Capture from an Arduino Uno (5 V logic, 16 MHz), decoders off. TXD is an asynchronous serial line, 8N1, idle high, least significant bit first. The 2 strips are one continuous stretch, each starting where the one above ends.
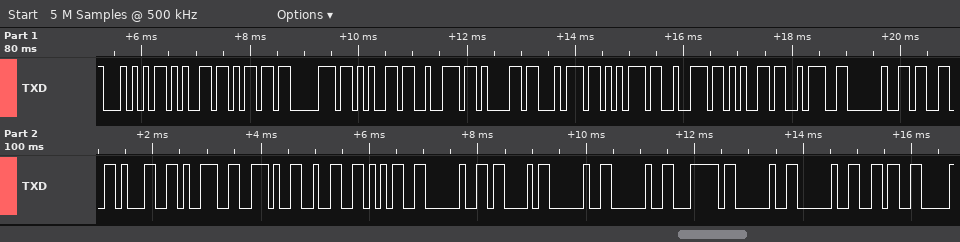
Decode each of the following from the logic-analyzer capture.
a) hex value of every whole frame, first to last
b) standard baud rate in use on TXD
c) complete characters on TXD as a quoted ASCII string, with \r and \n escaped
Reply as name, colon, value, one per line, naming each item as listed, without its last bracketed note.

hex value of every whole frame, first to last: 0x54 0x65 0x6D 0x70 0x65 0x72 0x61 0x74 0x75 0x72 0x65 0x3A 0x20 0x33 0x31 0x39 0x2E 0x32 0x35 0x20 0x43 0x20 0x20 0x7C 0x20 0x20 0x36
standard baud rate in use on TXD: 9600 baud
complete characters on TXD as a quoted ASCII string, with \r and \n escaped: "Temperature: 319.25 C  |  6"
